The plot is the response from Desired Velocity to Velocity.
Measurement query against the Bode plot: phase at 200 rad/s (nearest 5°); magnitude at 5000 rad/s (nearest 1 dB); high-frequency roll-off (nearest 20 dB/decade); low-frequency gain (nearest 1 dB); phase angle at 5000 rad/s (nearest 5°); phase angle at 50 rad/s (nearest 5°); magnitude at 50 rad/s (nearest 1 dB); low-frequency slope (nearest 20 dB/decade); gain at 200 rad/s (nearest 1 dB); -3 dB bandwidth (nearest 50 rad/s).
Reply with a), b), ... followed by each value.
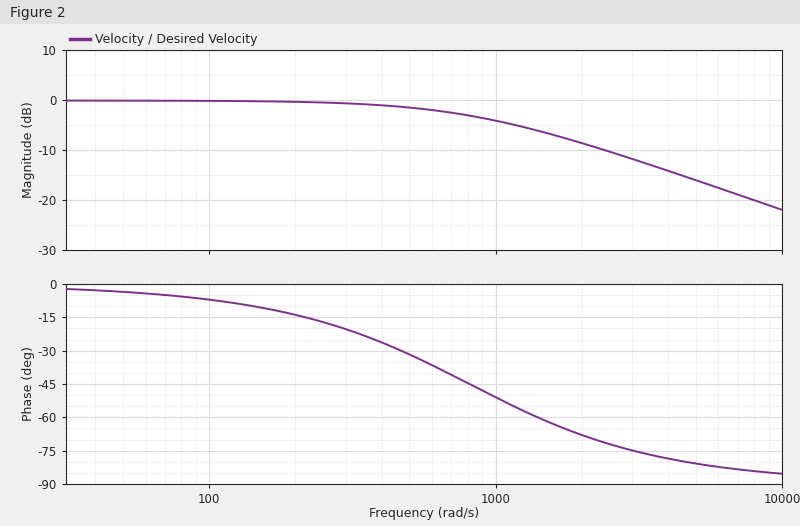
a) -15°
b) -16 dB
c) -20 dB/decade
d) 0 dB
e) -80°
f) -5°
g) 0 dB
h) 0 dB/decade
i) 0 dB
j) 800 rad/s
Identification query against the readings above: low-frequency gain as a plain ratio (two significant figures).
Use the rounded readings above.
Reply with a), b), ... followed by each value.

a) 1.0
